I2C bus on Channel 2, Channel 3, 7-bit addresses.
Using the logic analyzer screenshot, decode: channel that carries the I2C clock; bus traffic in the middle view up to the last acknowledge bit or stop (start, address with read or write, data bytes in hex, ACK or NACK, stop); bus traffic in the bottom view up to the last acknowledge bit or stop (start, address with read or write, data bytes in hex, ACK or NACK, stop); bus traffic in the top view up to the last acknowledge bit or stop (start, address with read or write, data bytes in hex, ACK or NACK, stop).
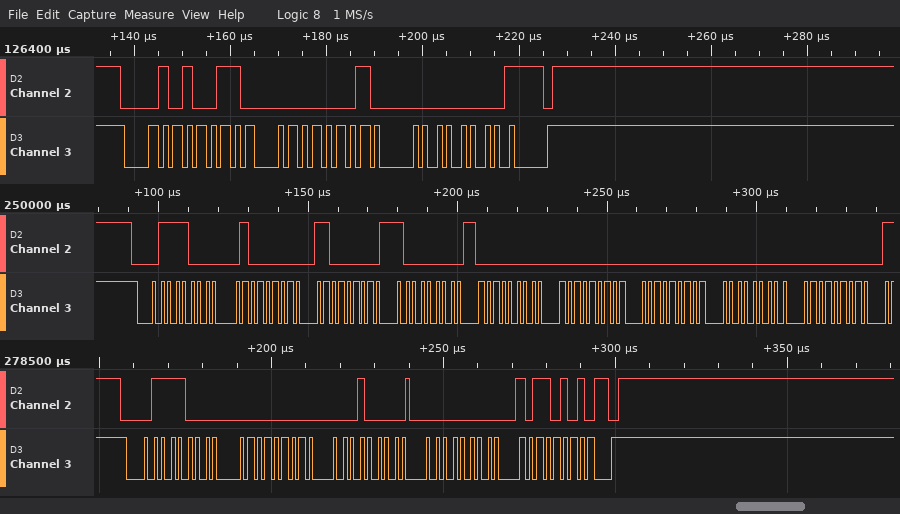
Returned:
Channel 3
start, address 3C write ACK, 40 ACK, C0 ACK, 80 ACK, 00 ACK, 00 ACK, 00 ACK, 00 ACK, 00 ACK
start, address 3C write ACK, 00 ACK, 10 ACK, 00 ACK, B5 ACK, stop
start, address 29 read ACK, 01 ACK, 00 NACK, stop
